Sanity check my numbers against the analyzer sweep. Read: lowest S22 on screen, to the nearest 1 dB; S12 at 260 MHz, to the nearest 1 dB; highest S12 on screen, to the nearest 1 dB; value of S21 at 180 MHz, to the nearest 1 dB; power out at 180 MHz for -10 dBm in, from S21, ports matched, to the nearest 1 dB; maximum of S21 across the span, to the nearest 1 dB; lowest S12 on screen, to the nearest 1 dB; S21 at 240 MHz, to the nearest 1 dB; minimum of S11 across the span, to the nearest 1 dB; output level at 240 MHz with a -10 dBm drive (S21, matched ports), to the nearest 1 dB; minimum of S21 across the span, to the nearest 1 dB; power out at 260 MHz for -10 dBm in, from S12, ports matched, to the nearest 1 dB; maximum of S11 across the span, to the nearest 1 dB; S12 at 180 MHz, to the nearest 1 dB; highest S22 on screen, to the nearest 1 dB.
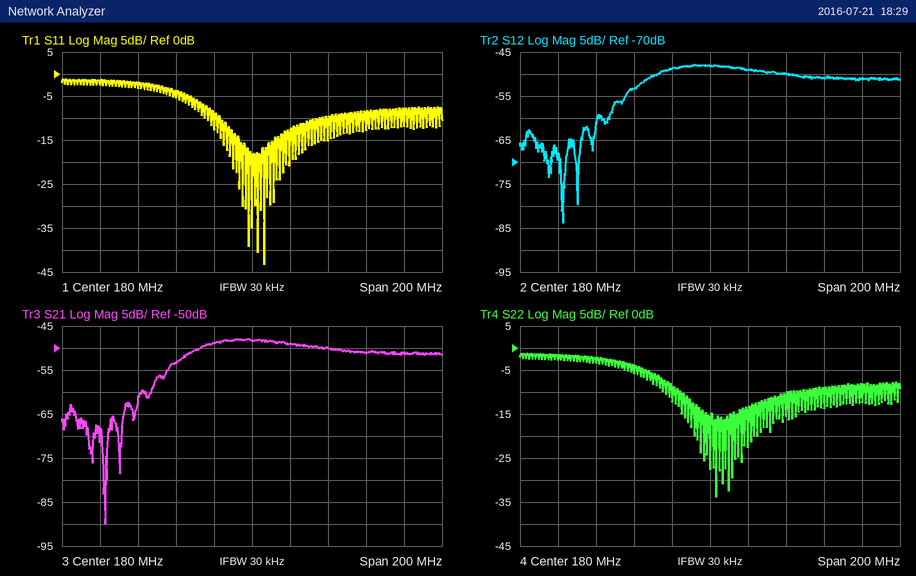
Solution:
-34 dB
-51 dB
-48 dB
-48 dB
-58 dBm
-48 dB
-84 dB
-51 dB
-43 dB
-61 dBm
-90 dB
-61 dBm
-1 dB
-48 dB
-1 dB
